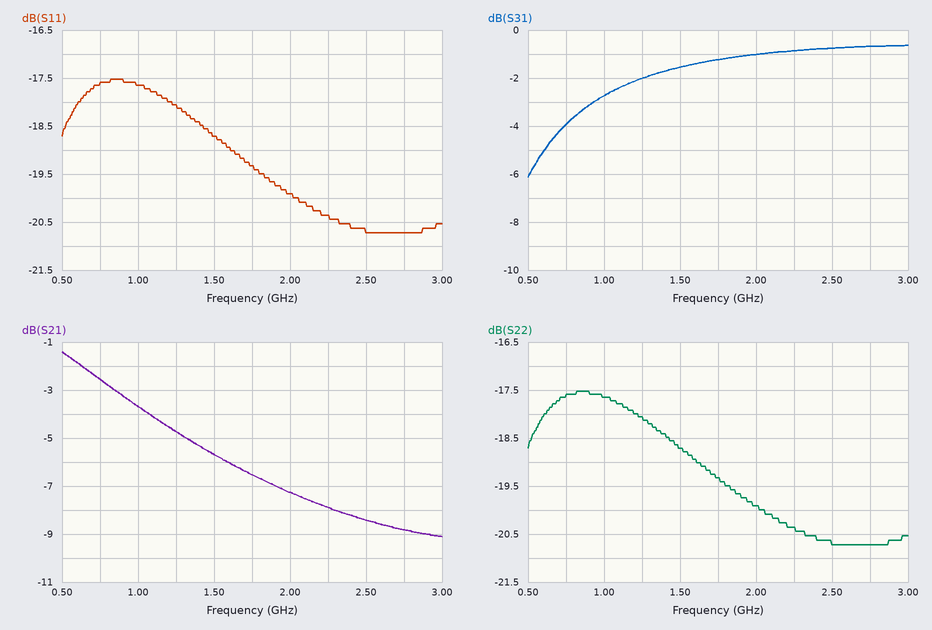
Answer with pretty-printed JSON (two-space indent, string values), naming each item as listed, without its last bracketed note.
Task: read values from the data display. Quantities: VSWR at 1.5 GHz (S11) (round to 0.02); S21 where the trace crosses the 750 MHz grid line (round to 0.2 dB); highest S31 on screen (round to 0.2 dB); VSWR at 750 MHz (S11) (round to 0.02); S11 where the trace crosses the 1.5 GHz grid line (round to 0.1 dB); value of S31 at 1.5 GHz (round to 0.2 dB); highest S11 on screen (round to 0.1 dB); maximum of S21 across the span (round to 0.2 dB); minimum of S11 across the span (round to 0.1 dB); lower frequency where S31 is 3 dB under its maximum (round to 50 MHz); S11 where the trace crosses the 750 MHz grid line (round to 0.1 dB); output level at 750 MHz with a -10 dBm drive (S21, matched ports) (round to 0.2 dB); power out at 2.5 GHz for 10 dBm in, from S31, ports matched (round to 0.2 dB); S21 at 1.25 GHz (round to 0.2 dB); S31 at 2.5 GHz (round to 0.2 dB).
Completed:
{
  "VSWR at 1.5 GHz (S11)": "1.26",
  "S21 where the trace crosses the 750 MHz grid line": "-2.6 dB",
  "highest S31 on screen": "-0.6 dB",
  "VSWR at 750 MHz (S11)": "1.30",
  "S11 where the trace crosses the 1.5 GHz grid line": "-18.7 dB",
  "value of S31 at 1.5 GHz": "-1.6 dB",
  "highest S11 on screen": "-17.5 dB",
  "maximum of S21 across the span": "-1.4 dB",
  "minimum of S11 across the span": "-20.7 dB",
  "lower frequency where S31 is 3 dB under its maximum": "800 MHz",
  "S11 where the trace crosses the 750 MHz grid line": "-17.6 dB",
  "output level at 750 MHz with a -10 dBm drive (S21, matched ports)": "-12.6 dBm",
  "power out at 2.5 GHz for 10 dBm in, from S31, ports matched": "9.2 dBm",
  "S21 at 1.25 GHz": "-4.8 dB",
  "S31 at 2.5 GHz": "-0.8 dB"
}
